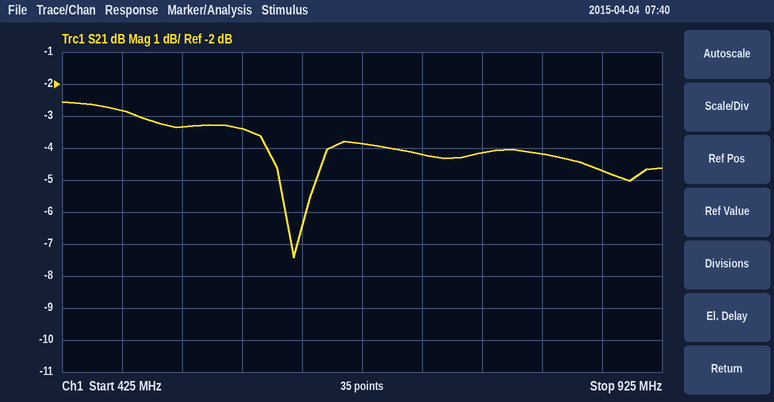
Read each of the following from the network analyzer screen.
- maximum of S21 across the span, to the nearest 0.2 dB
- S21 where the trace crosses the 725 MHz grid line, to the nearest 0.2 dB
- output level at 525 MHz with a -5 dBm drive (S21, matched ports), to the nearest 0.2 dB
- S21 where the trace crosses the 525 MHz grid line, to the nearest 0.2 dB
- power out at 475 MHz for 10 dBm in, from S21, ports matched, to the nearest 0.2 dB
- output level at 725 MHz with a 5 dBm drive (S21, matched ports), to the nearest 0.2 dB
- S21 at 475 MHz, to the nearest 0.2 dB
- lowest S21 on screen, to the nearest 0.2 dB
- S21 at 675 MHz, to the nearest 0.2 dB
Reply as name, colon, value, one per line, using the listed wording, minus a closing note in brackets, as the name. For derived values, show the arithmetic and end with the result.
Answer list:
maximum of S21 across the span, to the nearest 0.2 dB: -2.6 dB
S21 where the trace crosses the 725 MHz grid line, to the nearest 0.2 dB: -4.2 dB
output level at 525 MHz with a -5 dBm drive (S21, matched ports), to the nearest 0.2 dB: -5 dBm + (-3.4 dB) = -8.4 dBm
S21 where the trace crosses the 525 MHz grid line, to the nearest 0.2 dB: -3.4 dB
power out at 475 MHz for 10 dBm in, from S21, ports matched, to the nearest 0.2 dB: 10 dBm + (-2.8 dB) = 7.2 dBm
output level at 725 MHz with a 5 dBm drive (S21, matched ports), to the nearest 0.2 dB: 5 dBm + (-4.2 dB) = 0.8 dBm
S21 at 475 MHz, to the nearest 0.2 dB: -2.8 dB
lowest S21 on screen, to the nearest 0.2 dB: -7.4 dB
S21 at 675 MHz, to the nearest 0.2 dB: -3.8 dB
